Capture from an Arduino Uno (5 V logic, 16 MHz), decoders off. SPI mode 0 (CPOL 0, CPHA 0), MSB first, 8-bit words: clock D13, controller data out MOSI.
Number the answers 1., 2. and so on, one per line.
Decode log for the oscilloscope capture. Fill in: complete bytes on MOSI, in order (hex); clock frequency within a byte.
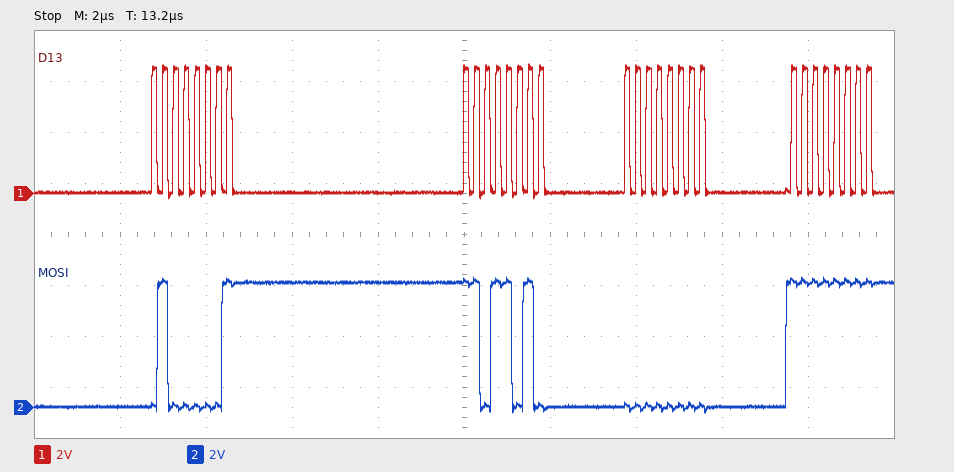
1. 41 DA 00 FF
2. 4 MHz
